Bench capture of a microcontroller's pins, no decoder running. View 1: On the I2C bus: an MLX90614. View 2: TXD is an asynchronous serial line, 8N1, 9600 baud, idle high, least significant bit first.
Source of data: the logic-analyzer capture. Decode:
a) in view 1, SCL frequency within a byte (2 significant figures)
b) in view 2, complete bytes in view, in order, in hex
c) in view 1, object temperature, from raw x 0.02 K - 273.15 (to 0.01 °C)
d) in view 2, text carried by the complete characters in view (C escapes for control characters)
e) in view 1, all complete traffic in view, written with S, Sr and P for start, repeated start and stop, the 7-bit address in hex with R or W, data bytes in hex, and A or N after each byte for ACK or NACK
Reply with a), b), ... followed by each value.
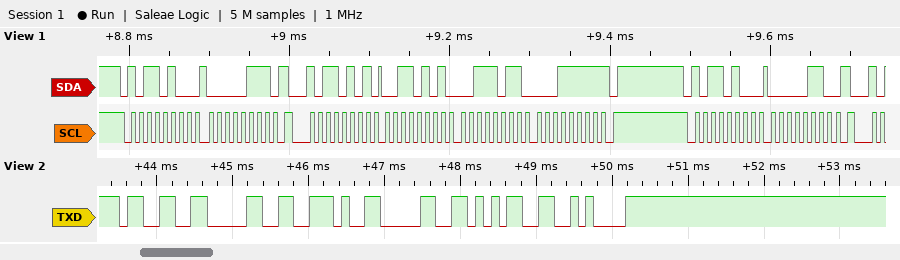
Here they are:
a) 100 kHz
b) 33 30 2E 30 35 0A
c) 29.99 °C
d) "30.05\n"
e) S 5AW A 07 A Sr 5AR A 35 A 3B A 1F N P S 5AW A 06 A
